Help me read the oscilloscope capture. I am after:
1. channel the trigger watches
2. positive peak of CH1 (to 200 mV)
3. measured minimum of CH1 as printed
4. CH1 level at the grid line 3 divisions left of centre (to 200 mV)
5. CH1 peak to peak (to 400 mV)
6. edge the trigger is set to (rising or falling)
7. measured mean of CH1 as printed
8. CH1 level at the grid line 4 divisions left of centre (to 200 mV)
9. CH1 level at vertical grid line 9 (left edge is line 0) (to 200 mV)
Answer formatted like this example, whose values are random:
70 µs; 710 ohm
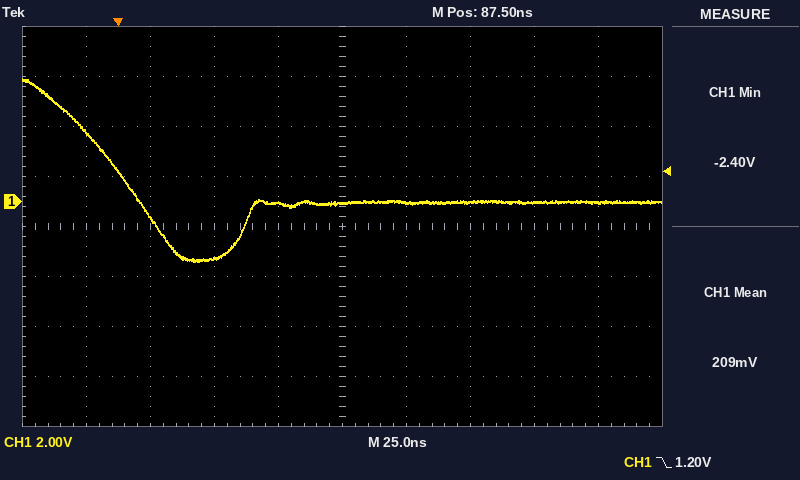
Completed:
CH1; 5.0 V; -2.40 V; -600 mV; 7.2 V; falling; 209 mV; 2.8 V; 0.0 V
